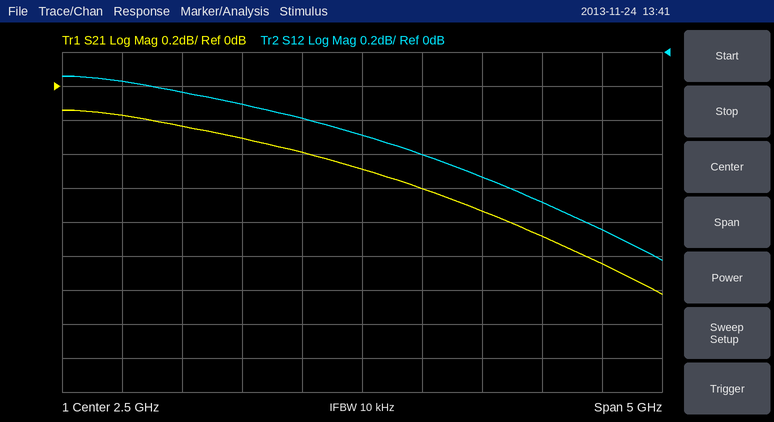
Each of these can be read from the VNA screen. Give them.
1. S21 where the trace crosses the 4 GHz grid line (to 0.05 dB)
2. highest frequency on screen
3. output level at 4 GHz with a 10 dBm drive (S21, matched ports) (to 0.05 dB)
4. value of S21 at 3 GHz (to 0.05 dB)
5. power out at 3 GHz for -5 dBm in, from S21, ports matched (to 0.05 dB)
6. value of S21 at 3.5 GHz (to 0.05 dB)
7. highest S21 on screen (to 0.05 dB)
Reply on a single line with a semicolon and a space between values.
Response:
-0.90 dB; 5 GHz; 9.10 dBm; -0.60 dB; -5.60 dBm; -0.75 dB; -0.15 dB
